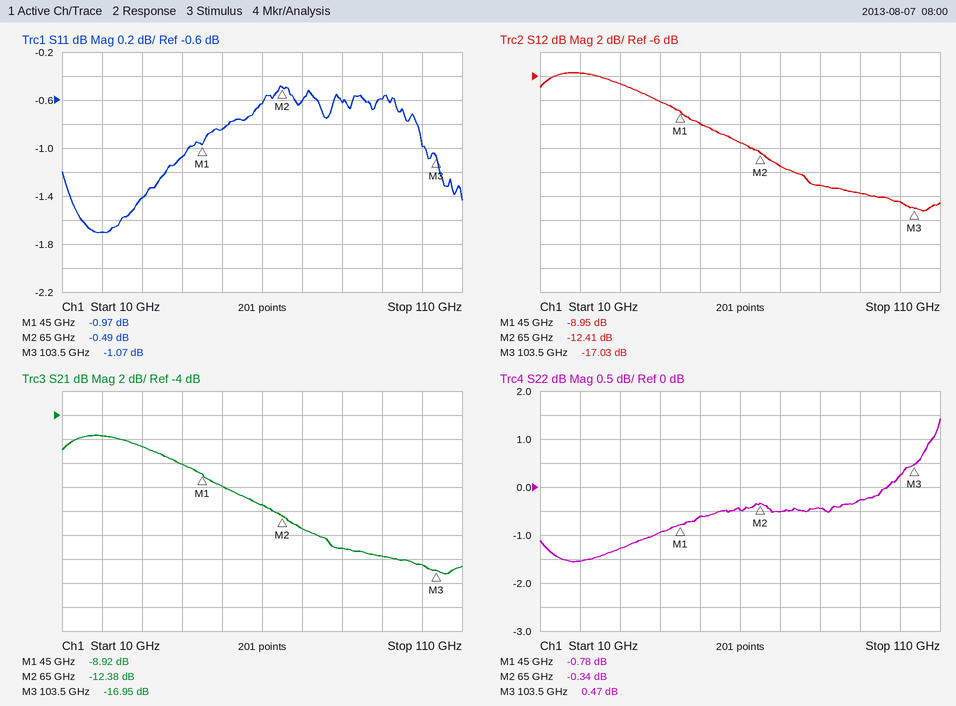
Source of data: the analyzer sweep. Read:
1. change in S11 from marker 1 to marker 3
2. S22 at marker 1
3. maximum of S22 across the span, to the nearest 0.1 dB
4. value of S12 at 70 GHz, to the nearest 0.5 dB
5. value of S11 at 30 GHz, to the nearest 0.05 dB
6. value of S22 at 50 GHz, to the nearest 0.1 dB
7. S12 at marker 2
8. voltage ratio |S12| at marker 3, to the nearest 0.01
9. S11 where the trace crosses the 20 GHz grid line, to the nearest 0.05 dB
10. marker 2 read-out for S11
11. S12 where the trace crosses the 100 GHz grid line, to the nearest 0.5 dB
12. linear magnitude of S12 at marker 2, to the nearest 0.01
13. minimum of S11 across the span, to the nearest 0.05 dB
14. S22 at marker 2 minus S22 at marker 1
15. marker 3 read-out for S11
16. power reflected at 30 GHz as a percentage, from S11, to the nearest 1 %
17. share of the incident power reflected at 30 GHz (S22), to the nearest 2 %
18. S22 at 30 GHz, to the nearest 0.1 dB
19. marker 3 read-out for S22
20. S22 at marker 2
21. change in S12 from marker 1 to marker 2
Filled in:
-0.10 dB
-0.78 dB
1.4 dB
-13.5 dB
-1.40 dB
-0.6 dB
-12.41 dB
0.14
-1.70 dB
-0.49 dB
-16.5 dB
0.24
-1.70 dB
0.44 dB
-1.07 dB
72 %
74 %
-1.3 dB
0.47 dB
-0.34 dB
-3.46 dB
